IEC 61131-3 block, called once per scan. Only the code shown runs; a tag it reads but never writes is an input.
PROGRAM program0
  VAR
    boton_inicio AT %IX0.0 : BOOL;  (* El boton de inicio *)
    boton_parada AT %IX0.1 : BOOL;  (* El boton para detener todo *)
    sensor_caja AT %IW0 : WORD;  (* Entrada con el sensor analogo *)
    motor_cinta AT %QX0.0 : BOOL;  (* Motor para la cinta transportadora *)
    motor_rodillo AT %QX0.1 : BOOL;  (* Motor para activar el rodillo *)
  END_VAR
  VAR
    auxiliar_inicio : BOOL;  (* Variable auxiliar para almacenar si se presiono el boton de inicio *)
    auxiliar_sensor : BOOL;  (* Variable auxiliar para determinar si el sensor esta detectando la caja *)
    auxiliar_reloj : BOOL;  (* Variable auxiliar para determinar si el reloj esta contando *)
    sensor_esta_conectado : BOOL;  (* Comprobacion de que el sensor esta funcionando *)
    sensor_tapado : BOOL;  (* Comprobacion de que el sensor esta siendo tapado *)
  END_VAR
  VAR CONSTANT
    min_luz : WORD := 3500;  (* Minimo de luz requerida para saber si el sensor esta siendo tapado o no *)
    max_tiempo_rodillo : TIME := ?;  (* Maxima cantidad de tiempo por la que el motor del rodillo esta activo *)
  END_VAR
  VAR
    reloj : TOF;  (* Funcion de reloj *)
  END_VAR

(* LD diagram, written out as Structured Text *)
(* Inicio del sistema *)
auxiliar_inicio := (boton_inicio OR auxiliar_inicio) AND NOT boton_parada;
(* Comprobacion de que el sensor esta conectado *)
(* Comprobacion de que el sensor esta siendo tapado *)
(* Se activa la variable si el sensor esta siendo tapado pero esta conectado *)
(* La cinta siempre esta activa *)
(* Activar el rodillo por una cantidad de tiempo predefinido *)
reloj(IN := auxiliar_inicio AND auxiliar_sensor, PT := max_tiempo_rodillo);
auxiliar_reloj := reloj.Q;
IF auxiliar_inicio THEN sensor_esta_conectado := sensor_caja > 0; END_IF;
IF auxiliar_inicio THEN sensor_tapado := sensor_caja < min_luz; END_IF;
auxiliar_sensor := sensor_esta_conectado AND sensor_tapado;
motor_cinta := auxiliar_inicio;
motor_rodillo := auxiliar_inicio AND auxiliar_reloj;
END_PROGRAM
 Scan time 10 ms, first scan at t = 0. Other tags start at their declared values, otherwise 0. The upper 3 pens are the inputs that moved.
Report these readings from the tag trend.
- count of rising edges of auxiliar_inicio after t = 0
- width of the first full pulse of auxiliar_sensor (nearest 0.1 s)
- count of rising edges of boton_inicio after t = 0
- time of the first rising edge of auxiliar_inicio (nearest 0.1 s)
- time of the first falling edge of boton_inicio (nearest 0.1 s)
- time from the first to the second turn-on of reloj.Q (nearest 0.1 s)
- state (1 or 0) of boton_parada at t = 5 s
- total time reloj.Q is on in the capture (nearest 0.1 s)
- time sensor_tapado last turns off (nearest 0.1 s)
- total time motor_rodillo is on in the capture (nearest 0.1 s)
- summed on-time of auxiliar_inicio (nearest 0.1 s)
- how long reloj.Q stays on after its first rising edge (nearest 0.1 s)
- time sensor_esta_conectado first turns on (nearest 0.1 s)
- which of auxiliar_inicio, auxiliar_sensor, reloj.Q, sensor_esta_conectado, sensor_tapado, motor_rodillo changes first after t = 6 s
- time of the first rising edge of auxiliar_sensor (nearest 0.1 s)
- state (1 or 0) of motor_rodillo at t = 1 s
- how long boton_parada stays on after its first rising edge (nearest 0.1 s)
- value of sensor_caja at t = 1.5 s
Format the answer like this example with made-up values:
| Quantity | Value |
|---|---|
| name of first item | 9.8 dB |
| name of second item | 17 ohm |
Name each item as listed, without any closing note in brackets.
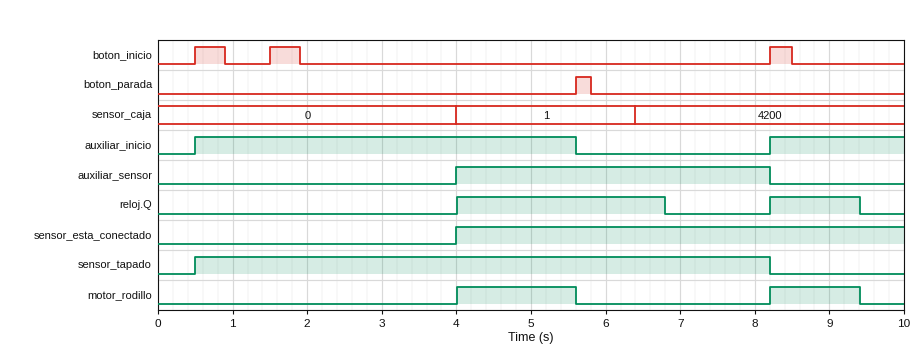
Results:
| Quantity | Value |
|---|---|
| count of rising edges of auxiliar_inicio after t = 0 | 2 |
| width of the first full pulse of auxiliar_sensor | 4.2 s |
| count of rising edges of boton_inicio after t = 0 | 3 |
| time of the first rising edge of auxiliar_inicio | 0.5 s |
| time of the first falling edge of boton_inicio | 0.9 s |
| time from the first to the second turn-on of reloj.Q | 4.2 s |
| state (1 or 0) of boton_parada at t = 5 s | 0 |
| total time reloj.Q is on in the capture | 4.0 s |
| time sensor_tapado last turns off | 8.2 s |
| total time motor_rodillo is on in the capture | 2.8 s |
| summed on-time of auxiliar_inicio | 6.9 s |
| how long reloj.Q stays on after its first rising edge | 2.8 s |
| time sensor_esta_conectado first turns on | 4.0 s |
| which of auxiliar_inicio, auxiliar_sensor, reloj.Q, sensor_esta_conectado, sensor_tapado, motor_rodillo changes first after t = 6 s | reloj.Q |
| time of the first rising edge of auxiliar_sensor | 4.0 s |
| state (1 or 0) of motor_rodillo at t = 1 s | 0 |
| how long boton_parada stays on after its first rising edge | 0.2 s |
| value of sensor_caja at t = 1.5 s | 0 |
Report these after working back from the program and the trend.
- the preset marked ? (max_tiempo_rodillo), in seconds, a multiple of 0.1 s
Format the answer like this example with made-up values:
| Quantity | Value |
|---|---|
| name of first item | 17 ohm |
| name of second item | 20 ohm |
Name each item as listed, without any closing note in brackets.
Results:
| Quantity | Value |
|---|---|
| the preset marked ? (max_tiempo_rodillo), in seconds, a multiple of 0.1 s | 1.2 s |
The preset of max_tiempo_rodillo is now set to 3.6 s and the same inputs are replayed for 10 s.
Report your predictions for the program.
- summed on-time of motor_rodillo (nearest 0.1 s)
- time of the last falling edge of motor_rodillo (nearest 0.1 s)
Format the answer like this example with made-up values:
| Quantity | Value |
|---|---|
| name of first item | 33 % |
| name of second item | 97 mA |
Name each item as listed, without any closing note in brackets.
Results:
| Quantity | Value |
|---|---|
| summed on-time of motor_rodillo | 3.4 s |
| time of the last falling edge of motor_rodillo | 5.6 s |
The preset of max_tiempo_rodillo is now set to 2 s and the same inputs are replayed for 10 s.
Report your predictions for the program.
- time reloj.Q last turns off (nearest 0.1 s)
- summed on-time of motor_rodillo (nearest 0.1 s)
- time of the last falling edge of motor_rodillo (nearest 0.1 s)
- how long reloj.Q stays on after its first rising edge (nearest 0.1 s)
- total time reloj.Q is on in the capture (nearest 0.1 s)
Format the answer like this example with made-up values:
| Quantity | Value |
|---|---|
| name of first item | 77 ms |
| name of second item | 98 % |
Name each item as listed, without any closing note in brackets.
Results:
| Quantity | Value |
|---|---|
| time reloj.Q last turns off | 7.6 s |
| summed on-time of motor_rodillo | 3.4 s |
| time of the last falling edge of motor_rodillo | 5.6 s |
| how long reloj.Q stays on after its first rising edge | 3.6 s |
| total time reloj.Q is on in the capture | 5.4 s |
